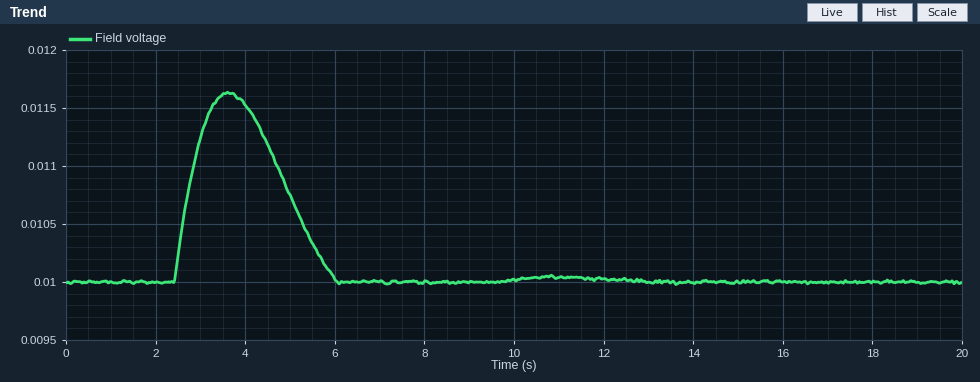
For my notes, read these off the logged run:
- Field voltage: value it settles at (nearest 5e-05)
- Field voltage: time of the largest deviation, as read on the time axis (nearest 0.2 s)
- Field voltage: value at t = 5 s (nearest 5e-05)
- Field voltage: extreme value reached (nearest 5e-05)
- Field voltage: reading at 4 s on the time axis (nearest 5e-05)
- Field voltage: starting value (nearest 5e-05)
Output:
0.01000
3.6 s
0.01075
0.01165
0.01155
0.01000
